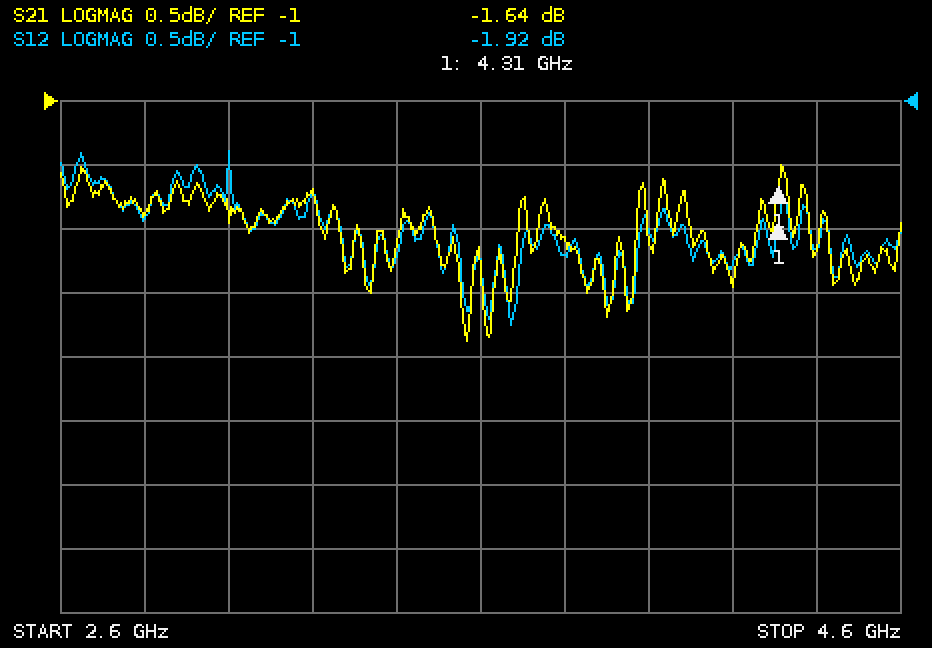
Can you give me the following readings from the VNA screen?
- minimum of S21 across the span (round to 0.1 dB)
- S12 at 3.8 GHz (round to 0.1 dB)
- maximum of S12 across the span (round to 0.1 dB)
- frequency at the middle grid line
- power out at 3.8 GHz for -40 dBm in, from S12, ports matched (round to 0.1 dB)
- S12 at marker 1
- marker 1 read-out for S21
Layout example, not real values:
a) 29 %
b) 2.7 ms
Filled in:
a) -2.9 dB
b) -2.2 dB
c) -1.4 dB
d) 3.6 GHz
e) -42.2 dBm
f) -1.92 dB
g) -1.64 dB
